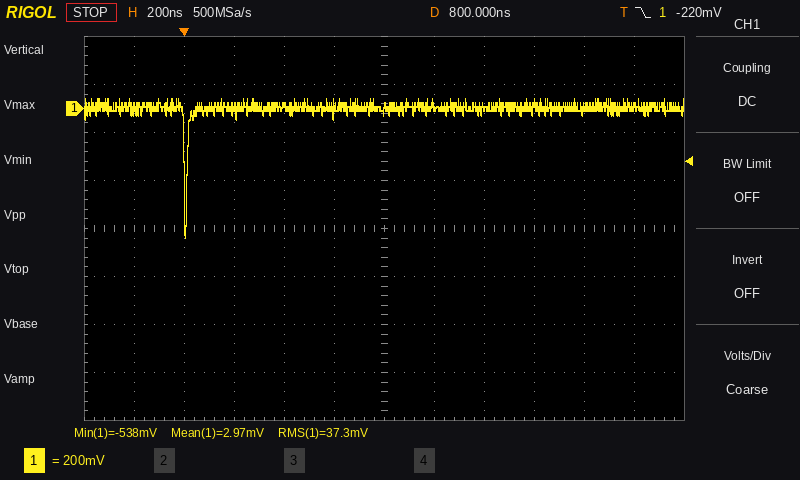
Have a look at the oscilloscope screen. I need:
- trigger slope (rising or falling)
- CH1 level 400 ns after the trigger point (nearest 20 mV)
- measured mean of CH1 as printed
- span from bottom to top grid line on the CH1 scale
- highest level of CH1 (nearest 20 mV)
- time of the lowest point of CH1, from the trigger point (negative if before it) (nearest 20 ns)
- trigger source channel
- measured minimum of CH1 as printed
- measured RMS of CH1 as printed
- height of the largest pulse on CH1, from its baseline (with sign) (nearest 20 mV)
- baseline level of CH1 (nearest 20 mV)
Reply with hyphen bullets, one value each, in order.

- falling
- 0 mV
- 2.97 mV
- 1.6 V
- 40 mV
- 0 ns
- CH1
- -538 mV
- 37.3 mV
- -540 mV
- 0 mV
